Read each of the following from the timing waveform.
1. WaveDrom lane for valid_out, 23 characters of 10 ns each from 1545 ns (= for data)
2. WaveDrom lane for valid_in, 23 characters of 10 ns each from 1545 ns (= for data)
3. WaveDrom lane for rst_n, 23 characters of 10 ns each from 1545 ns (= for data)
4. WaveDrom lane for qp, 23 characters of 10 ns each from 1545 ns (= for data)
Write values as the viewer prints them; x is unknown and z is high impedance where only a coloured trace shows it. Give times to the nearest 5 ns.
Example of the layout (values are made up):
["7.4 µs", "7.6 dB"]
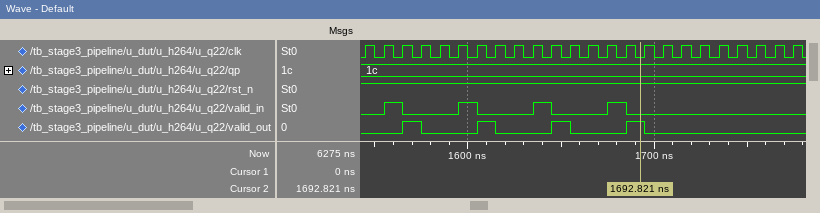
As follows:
["{name: 'valid_out', wave: '0.10..10..10..10.......'}", "{name: 'valid_in', wave: '010..10..10..10........'}", "{name: 'rst_n', wave: '1......................'}", "{name: 'qp', wave: '=......................', data: '1c'}"]
